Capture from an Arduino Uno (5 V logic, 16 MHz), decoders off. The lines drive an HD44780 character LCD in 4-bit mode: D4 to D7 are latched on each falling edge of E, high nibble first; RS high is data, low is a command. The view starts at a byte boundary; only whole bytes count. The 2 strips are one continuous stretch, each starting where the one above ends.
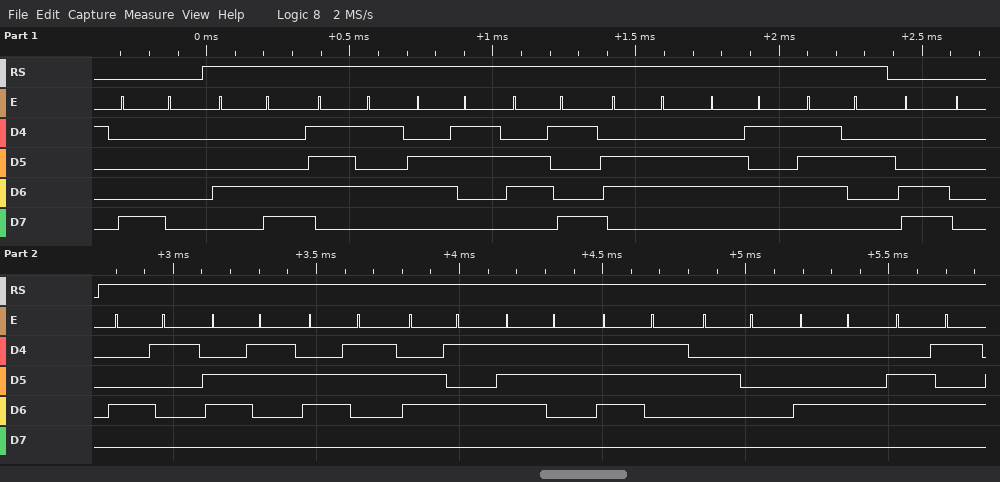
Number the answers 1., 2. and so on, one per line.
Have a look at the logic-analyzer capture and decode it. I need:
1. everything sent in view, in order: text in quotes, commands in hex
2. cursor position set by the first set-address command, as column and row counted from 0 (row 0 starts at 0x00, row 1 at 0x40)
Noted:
1. 0x80 "Lucifer" 0xC0 "Access De"
2. column 0, row 0
